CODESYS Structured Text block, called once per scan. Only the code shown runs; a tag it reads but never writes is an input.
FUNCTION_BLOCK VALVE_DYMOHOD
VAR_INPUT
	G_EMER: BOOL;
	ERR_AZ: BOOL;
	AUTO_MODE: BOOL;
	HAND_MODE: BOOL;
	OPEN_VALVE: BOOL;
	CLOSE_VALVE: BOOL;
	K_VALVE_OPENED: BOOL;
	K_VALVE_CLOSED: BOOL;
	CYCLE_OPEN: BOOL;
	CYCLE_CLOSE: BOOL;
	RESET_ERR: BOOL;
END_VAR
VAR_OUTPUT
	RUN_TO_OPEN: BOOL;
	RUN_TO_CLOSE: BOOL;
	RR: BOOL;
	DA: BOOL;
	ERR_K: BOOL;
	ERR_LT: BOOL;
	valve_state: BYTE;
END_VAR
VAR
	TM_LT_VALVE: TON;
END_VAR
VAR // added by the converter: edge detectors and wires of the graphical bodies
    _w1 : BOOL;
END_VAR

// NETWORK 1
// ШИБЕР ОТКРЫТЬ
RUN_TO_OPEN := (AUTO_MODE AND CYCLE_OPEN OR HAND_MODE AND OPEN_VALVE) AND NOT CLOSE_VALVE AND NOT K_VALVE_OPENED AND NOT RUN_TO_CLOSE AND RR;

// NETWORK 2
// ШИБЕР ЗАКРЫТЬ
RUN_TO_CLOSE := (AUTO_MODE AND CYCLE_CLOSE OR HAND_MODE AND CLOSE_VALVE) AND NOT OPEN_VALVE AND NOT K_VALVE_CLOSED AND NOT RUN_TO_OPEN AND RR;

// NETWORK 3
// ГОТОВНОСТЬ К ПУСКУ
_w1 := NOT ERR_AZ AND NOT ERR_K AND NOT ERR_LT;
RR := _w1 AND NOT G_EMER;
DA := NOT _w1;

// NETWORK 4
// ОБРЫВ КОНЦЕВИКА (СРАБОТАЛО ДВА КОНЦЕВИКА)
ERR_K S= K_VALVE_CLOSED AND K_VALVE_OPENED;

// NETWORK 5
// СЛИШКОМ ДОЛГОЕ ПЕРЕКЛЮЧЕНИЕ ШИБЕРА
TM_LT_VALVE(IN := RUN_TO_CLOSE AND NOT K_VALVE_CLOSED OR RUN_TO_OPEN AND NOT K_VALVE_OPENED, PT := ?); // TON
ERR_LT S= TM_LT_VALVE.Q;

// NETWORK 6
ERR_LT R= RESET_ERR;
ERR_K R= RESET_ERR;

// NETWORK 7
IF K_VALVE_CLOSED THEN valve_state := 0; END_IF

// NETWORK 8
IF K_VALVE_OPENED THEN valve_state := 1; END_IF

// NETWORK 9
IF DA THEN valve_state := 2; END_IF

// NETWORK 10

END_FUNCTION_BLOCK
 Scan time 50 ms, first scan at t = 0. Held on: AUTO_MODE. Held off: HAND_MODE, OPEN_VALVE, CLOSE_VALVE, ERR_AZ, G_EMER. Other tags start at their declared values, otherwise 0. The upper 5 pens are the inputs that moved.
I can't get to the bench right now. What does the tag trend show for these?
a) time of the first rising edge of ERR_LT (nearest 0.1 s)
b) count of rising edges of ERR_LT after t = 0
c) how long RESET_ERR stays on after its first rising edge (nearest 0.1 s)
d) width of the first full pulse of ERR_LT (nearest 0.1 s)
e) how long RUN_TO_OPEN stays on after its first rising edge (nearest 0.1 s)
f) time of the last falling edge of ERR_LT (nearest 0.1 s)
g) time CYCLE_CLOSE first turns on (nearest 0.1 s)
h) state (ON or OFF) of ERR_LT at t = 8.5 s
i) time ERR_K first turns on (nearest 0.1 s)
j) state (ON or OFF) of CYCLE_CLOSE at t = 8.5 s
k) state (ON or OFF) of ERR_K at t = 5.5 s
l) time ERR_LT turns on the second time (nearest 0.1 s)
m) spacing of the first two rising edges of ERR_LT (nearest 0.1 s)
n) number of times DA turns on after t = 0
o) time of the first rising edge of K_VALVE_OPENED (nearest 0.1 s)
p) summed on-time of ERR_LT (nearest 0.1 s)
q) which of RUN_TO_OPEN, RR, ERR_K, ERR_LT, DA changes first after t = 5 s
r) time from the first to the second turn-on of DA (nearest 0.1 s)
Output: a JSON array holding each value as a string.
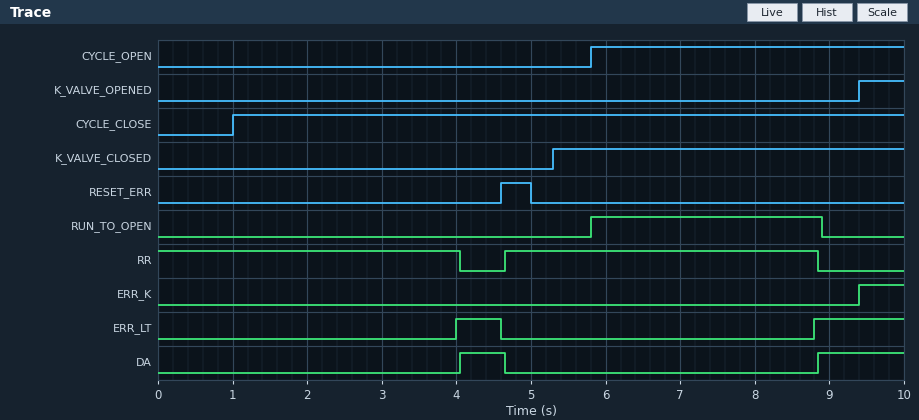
["4.0 s", "2", "0.4 s", "0.6 s", "3.1 s", "4.6 s", "1.0 s", "OFF", "9.4 s", "ON", "OFF", "8.8 s", "4.8 s", "2", "9.4 s", "1.8 s", "RUN_TO_OPEN", "4.8 s"]
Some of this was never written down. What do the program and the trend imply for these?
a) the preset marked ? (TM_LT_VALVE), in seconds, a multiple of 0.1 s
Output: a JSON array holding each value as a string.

["3.0 s"]
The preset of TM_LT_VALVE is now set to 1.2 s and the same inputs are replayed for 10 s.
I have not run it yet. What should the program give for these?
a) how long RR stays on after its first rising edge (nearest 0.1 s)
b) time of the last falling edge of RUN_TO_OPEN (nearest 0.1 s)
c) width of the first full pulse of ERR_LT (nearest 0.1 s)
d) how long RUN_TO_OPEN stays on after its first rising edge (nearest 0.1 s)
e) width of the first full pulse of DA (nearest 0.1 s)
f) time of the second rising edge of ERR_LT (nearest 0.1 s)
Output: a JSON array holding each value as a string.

["2.4 s", "7.1 s", "2.4 s", "1.3 s", "2.4 s", "7.0 s"]
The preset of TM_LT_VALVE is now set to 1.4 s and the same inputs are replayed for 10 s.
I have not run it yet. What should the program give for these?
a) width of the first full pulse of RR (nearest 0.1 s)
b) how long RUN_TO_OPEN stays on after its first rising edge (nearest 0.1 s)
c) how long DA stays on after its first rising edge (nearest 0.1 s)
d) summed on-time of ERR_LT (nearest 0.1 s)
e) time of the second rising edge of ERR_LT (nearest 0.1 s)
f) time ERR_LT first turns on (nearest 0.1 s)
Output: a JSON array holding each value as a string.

["2.6 s", "1.5 s", "2.2 s", "5.0 s", "7.2 s", "2.4 s"]
